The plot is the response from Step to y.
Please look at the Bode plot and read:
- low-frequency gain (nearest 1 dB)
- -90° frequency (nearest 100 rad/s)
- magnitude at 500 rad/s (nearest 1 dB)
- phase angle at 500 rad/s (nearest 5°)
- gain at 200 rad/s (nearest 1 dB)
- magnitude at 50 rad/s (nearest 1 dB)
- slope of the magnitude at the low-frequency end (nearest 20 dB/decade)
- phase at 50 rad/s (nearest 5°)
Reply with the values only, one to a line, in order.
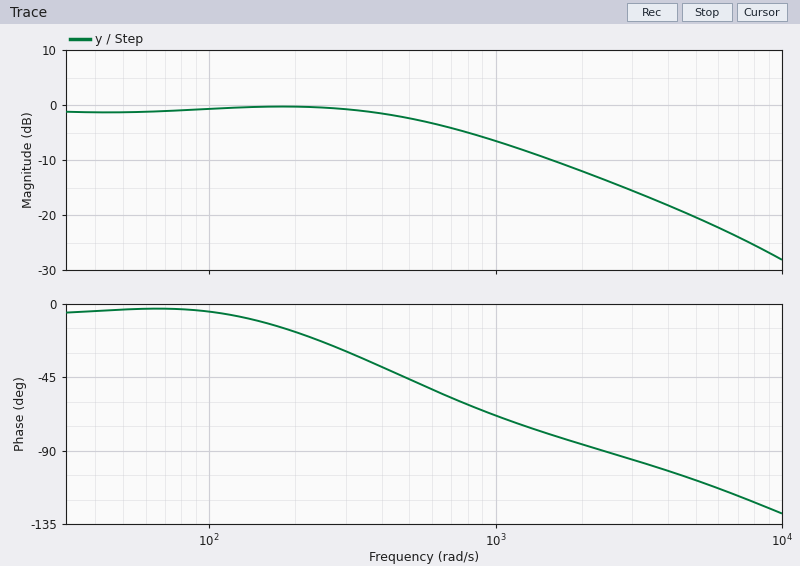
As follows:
-1 dB
2400 rad/s
-2 dB
-45°
0 dB
-1 dB
0 dB/decade
-5°
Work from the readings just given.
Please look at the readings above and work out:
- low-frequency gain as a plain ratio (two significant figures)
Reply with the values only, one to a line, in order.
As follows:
0.89
